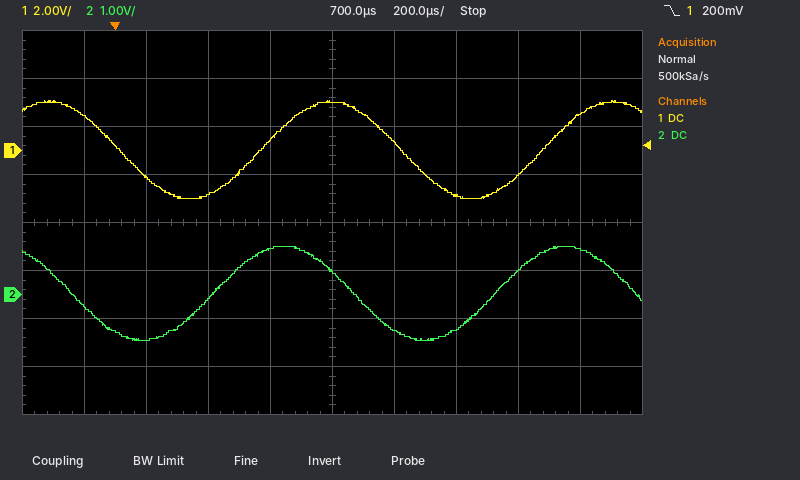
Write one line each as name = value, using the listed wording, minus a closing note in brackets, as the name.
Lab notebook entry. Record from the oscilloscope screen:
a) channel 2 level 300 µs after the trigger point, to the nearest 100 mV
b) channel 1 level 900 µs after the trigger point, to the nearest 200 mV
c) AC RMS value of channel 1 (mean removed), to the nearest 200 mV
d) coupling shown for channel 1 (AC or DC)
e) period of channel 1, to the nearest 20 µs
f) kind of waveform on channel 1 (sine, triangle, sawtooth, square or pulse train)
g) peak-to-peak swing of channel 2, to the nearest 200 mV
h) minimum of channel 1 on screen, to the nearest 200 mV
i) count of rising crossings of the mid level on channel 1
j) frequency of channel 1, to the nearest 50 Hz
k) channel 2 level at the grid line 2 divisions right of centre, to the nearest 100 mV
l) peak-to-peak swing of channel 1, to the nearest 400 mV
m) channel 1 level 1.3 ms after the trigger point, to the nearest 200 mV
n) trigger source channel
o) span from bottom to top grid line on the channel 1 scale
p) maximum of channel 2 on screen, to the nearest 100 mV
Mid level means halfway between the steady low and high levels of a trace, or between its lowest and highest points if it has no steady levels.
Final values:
channel 2 level 300 µs after the trigger point, to the nearest 100 mV = -100 mV
channel 1 level 900 µs after the trigger point, to the nearest 200 mV = 400 mV
AC RMS value of channel 1 (mean removed), to the nearest 200 mV = 1.4 V
coupling shown for channel 1 = DC
period of channel 1, to the nearest 20 µs = 900 µs
kind of waveform on channel 1 = sine
peak-to-peak swing of channel 2, to the nearest 200 mV = 2.0 V
minimum of channel 1 on screen, to the nearest 200 mV = -2.0 V
count of rising crossings of the mid level on channel 1 = 2
frequency of channel 1, to the nearest 50 Hz = 1.10 kHz
channel 2 level at the grid line 2 divisions right of centre, to the nearest 100 mV = -700 mV
peak-to-peak swing of channel 1, to the nearest 400 mV = 4.0 V
channel 1 level 1.3 ms after the trigger point, to the nearest 200 mV = -1.0 V
trigger source channel = channel 1
span from bottom to top grid line on the channel 1 scale = 16 V
maximum of channel 2 on screen, to the nearest 100 mV = 1.0 V
